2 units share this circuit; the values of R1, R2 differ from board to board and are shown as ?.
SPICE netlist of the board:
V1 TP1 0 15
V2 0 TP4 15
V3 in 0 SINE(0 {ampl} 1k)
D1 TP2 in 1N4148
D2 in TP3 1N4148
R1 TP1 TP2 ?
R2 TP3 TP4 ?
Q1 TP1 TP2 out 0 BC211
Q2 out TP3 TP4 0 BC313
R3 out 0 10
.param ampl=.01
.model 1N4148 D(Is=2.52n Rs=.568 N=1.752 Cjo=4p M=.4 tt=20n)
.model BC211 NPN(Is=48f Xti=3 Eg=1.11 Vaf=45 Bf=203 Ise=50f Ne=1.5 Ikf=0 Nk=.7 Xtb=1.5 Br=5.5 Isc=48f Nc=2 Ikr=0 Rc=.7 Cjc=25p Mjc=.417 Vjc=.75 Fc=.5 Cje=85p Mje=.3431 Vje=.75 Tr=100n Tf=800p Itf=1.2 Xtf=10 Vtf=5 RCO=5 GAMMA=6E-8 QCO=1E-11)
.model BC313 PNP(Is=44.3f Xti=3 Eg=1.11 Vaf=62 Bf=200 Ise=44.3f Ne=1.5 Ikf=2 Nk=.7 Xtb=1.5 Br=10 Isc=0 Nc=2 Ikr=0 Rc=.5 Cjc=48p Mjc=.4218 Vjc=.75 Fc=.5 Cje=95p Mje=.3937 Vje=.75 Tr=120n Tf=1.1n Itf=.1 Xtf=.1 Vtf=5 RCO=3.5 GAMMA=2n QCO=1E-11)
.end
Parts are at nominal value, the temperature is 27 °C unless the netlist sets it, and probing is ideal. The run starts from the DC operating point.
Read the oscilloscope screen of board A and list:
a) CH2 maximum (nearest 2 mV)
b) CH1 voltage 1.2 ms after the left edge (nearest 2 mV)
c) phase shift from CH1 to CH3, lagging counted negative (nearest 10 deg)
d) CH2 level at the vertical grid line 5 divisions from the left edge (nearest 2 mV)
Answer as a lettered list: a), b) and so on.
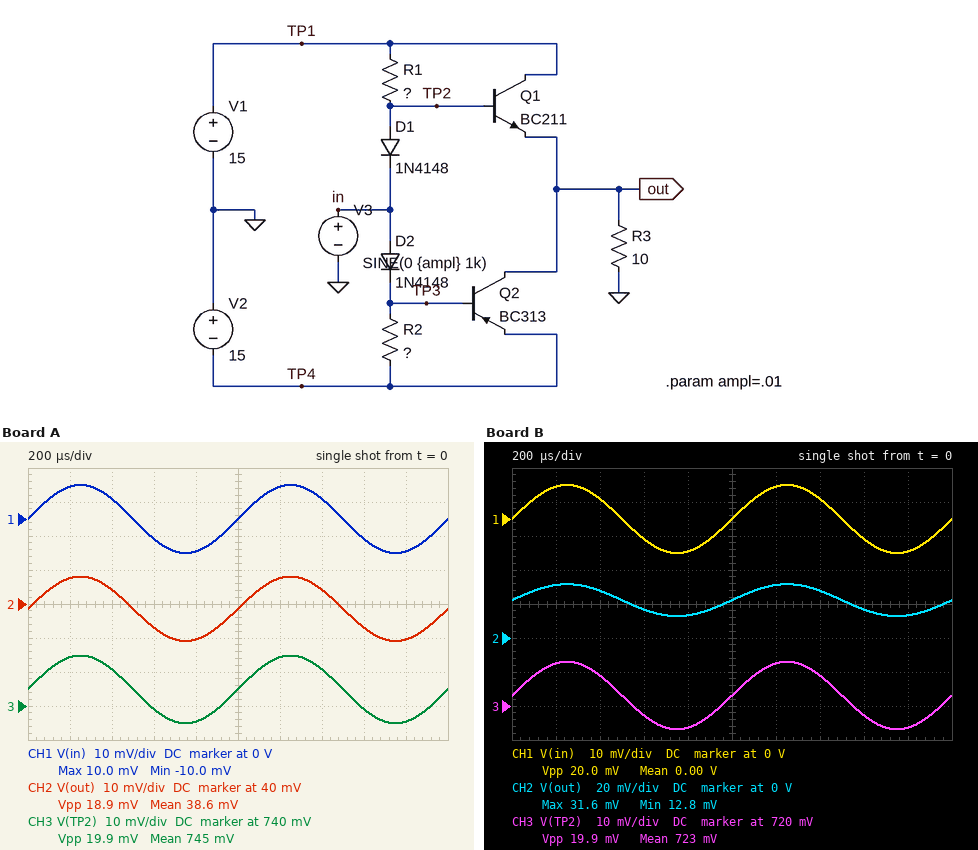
a) 48 mV
b) 10 mV
c) 0 deg
d) 38 mV
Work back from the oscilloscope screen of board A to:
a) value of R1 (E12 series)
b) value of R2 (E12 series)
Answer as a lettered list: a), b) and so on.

a) 560 Ω
b) 150 Ω
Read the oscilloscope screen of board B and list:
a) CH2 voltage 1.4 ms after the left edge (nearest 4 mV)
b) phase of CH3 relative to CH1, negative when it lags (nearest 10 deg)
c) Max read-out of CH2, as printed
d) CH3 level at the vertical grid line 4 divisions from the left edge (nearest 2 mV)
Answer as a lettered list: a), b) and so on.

a) 28 mV
b) 0 deg
c) 31.6 mV
d) 714 mV
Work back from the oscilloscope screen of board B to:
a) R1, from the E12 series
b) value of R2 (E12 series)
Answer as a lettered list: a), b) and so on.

a) 820 Ω
b) 180 Ω
